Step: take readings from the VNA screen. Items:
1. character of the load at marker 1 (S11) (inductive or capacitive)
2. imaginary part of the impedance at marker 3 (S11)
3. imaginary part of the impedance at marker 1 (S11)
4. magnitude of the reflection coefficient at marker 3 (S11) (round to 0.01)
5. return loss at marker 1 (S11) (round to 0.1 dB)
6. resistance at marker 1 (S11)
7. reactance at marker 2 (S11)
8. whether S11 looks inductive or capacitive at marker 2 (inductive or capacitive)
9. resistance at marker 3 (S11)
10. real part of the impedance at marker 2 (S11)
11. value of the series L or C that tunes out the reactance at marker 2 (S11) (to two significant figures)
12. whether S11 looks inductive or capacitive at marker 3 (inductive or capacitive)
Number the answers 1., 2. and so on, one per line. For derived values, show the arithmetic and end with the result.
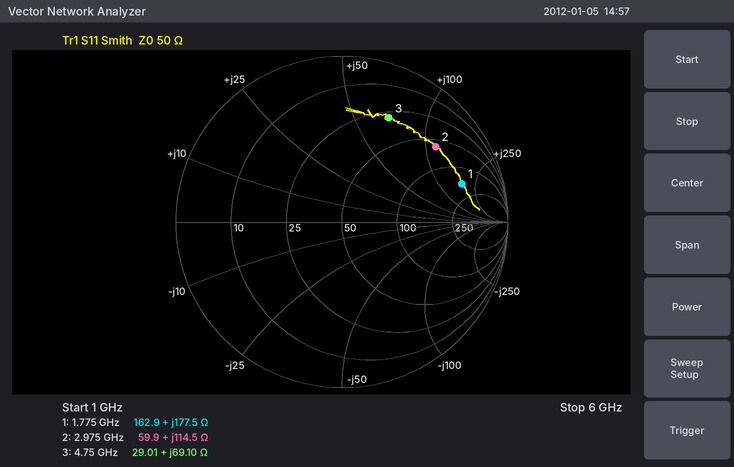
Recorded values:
1. inductive
2. +69.10 Ω
3. +177.5 Ω
4. 0.69
5. 2.4 dB
6. 162.9 Ω
7. +114.5 Ω
8. inductive
9. 29.01 Ω
10. 59.9 Ω
11. C = 1/(2π × 2.975 GHz × 114.5 Ω) ≈ 467 fF, so 470 fF to two significant figures
12. inductive
